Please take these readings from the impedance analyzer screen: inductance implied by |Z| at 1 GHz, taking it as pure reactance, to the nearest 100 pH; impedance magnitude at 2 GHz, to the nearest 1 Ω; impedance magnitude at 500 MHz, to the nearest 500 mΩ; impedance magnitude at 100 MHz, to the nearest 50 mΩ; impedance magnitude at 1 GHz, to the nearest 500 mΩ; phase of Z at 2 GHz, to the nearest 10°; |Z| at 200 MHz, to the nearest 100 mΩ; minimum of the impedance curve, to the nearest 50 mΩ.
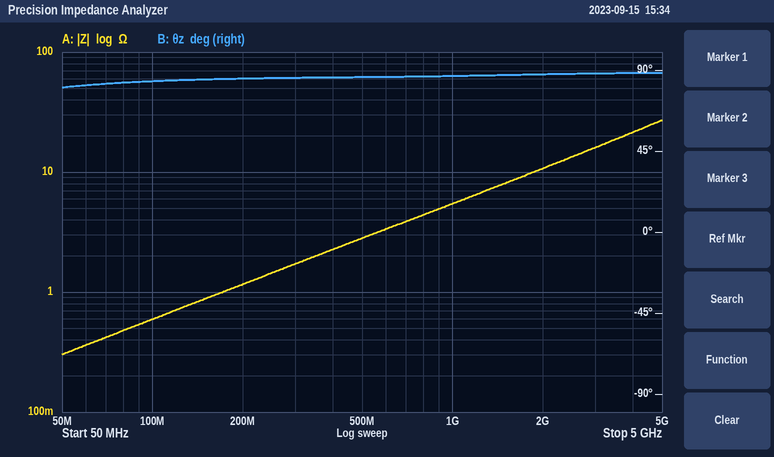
900 pH
11 Ω
3.0 Ω
600 mΩ
5.5 Ω
90°
1.2 Ω
300 mΩ
